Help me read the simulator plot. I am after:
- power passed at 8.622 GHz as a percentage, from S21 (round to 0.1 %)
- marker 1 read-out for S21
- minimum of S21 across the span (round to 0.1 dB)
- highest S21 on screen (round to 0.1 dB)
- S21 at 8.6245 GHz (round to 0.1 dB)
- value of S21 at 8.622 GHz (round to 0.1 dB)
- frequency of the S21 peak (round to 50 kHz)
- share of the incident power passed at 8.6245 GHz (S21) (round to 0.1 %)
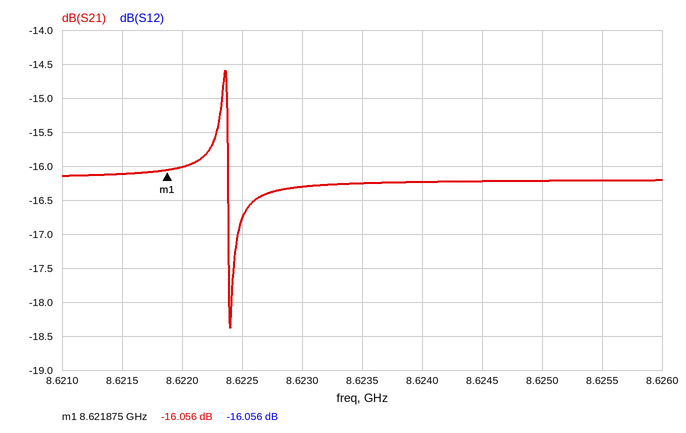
2.5 %
-16.056 dB
-18.4 dB
-14.6 dB
-16.2 dB
-16.0 dB
8.62235 GHz
2.4 %
